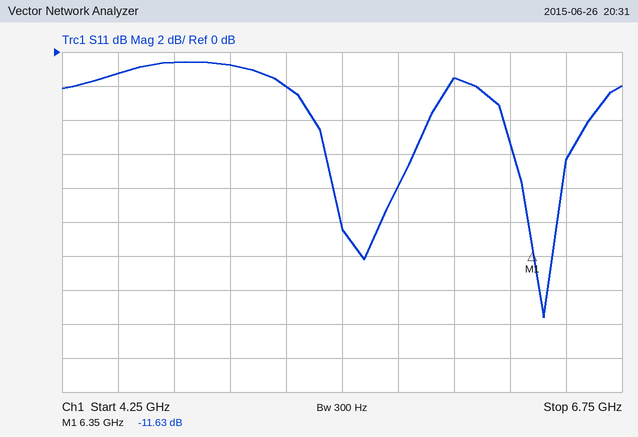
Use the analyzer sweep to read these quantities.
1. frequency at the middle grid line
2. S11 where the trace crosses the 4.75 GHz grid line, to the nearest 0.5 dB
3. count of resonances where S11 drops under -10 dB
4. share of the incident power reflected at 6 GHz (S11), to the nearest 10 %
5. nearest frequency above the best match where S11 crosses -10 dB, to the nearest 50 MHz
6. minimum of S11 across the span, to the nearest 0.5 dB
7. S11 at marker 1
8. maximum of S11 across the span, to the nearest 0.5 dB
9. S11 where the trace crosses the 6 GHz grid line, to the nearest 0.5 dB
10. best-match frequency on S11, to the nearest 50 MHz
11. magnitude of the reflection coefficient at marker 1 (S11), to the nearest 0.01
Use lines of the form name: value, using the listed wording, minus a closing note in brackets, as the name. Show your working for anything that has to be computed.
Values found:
frequency at the middle grid line: 5.5 GHz
S11 where the trace crosses the 4.75 GHz grid line, to the nearest 0.5 dB: -0.5 dB
count of resonances where S11 drops under -10 dB: 2
share of the incident power reflected at 6 GHz (S11), to the nearest 10 %: 10^(-1.5/10) ≈ 70.8 %, so 70 % to the nearest 10 %
nearest frequency above the best match where S11 crosses -10 dB, to the nearest 50 MHz: 6.45 GHz
minimum of S11 across the span, to the nearest 0.5 dB: -15.5 dB
S11 at marker 1: -11.63 dB
maximum of S11 across the span, to the nearest 0.5 dB: -0.5 dB
S11 where the trace crosses the 6 GHz grid line, to the nearest 0.5 dB: -1.5 dB
best-match frequency on S11, to the nearest 50 MHz: 6.40 GHz
magnitude of the reflection coefficient at marker 1 (S11), to the nearest 0.01: 10^(-11.63/20) ≈ 0.26
